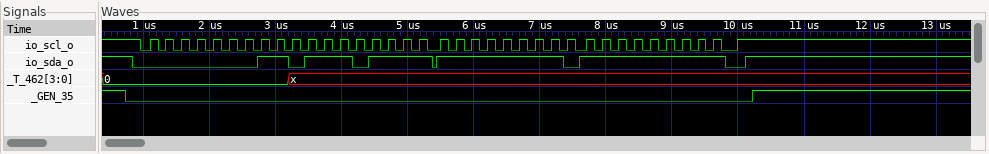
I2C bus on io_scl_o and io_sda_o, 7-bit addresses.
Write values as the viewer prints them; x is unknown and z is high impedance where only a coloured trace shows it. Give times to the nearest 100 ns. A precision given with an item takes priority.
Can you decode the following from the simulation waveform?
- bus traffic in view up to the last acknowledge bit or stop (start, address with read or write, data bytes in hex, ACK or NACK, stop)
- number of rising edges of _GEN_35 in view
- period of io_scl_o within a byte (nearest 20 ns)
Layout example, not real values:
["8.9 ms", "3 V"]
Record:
["start, address 00 read NACK, 77 NACK, FF ACK, FF NACK, stop", "1", "240 ns"]
